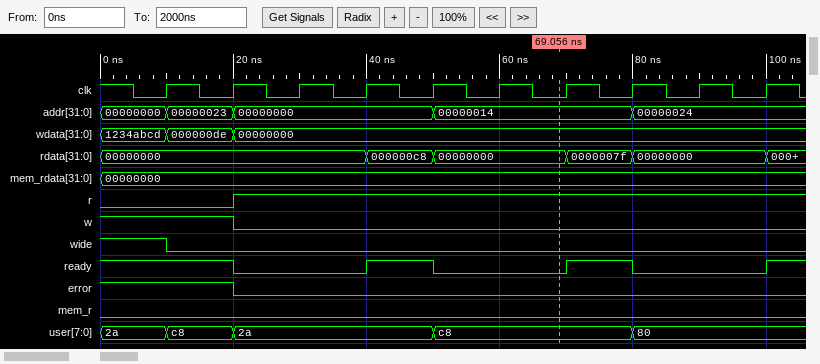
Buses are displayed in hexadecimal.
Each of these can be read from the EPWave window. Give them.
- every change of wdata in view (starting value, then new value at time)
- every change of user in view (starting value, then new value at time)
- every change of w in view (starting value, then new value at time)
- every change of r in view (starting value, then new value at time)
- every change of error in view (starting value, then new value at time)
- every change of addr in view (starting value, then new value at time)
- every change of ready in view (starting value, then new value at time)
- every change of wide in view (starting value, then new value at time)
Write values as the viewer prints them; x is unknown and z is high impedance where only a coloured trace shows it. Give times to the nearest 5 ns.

1234abcd, 000000de at 10 ns, 00000000 at 20 ns
2a, c8 at 10 ns, 2a at 20 ns, c8 at 50 ns, 80 at 80 ns
1, 0 at 20 ns
0, 1 at 20 ns
1, 0 at 20 ns
00000000, 00000023 at 10 ns, 00000000 at 20 ns, 00000014 at 50 ns, 00000024 at 80 ns
1, 0 at 20 ns, 1 at 40 ns, 0 at 50 ns, 1 at 70 ns, 0 at 80 ns, 1 at 100 ns
1, 0 at 10 ns
